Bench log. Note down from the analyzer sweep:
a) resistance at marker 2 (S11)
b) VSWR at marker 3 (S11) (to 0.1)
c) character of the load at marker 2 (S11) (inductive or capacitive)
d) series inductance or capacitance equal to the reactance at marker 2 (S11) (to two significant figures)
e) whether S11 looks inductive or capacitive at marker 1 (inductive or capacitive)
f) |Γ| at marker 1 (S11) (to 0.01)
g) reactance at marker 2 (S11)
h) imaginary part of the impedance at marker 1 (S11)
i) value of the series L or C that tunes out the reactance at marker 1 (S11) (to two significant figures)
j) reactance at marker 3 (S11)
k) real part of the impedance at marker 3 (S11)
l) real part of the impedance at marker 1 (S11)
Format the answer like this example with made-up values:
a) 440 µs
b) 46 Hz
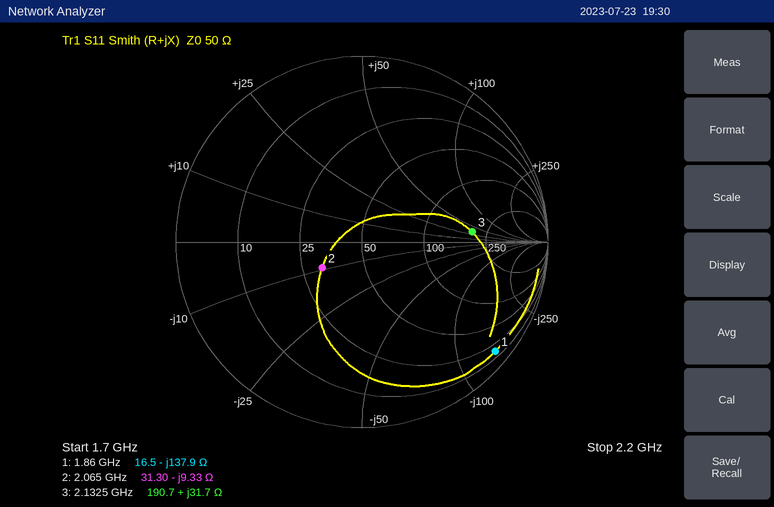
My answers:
a) 31.30 Ω
b) 3.9
c) capacitive
d) 8.3 pF
e) capacitive
f) 0.93
g) -9.33 Ω
h) -137.9 Ω
i) 12 nH
j) +31.7 Ω
k) 190.7 Ω
l) 16.5 Ω
